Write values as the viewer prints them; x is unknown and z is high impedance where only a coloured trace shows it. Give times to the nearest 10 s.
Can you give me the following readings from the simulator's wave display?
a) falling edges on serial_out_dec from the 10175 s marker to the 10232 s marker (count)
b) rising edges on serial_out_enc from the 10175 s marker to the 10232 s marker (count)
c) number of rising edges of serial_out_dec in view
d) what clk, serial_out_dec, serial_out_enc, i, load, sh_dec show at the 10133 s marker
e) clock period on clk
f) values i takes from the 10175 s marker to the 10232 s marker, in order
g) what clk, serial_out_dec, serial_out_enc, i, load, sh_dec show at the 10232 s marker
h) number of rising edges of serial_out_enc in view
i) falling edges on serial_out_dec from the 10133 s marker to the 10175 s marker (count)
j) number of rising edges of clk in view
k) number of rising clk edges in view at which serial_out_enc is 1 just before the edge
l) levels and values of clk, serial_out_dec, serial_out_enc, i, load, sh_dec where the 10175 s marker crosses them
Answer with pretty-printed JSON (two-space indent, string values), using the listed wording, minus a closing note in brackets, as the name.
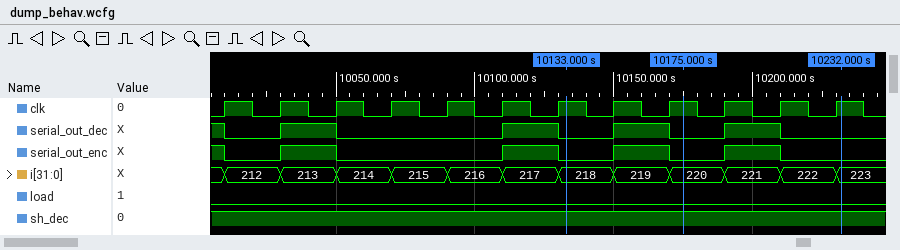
{
  "falling edges on serial_out_dec from the 10175 s marker to the 10232 s marker": "1",
  "rising edges on serial_out_enc from the 10175 s marker to the 10232 s marker": "1",
  "number of rising edges of serial_out_dec in view": "4",
  "what clk, serial_out_dec, serial_out_enc, i, load, sh_dec show at the 10133 s marker": "clk=1, serial_out_dec=0, serial_out_enc=0, i=218, load=0, sh_dec=1",
  "clock period on clk": "20 s",
  "values i takes from the 10175 s marker to the 10232 s marker, in order": "220, 221, 222, 223",
  "what clk, serial_out_dec, serial_out_enc, i, load, sh_dec show at the 10232 s marker": "clk=1, serial_out_dec=0, serial_out_enc=0, i=223, load=0, sh_dec=1",
  "number of rising edges of serial_out_enc in view": "4",
  "falling edges on serial_out_dec from the 10133 s marker to the 10175 s marker": "1",
  "number of rising edges of clk in view": "12",
  "number of rising clk edges in view at which serial_out_enc is 1 just before the edge": "5",
  "levels and values of clk, serial_out_dec, serial_out_enc, i, load, sh_dec where the 10175 s marker crosses them": "clk=1, serial_out_dec=0, serial_out_enc=0, i=220, load=0, sh_dec=1"
}
